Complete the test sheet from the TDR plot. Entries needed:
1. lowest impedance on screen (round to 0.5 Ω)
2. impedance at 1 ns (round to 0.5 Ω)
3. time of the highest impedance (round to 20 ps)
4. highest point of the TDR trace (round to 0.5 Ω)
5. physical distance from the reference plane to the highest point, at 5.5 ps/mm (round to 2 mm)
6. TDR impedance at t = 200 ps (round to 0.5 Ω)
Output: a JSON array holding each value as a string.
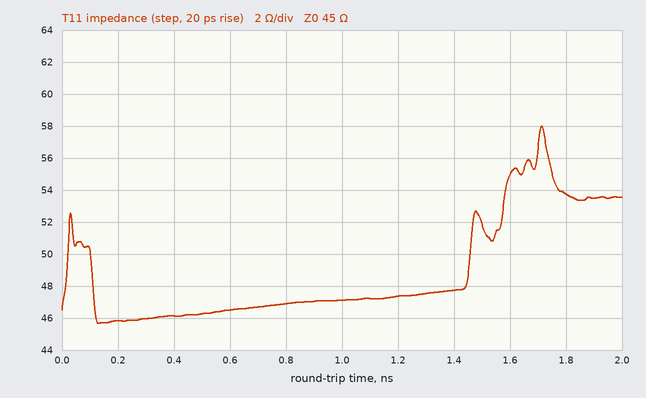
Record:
["45.5 Ω", "47.0 Ω", "1.72 ns", "58.0 Ω", "156 mm", "46.0 Ω"]
